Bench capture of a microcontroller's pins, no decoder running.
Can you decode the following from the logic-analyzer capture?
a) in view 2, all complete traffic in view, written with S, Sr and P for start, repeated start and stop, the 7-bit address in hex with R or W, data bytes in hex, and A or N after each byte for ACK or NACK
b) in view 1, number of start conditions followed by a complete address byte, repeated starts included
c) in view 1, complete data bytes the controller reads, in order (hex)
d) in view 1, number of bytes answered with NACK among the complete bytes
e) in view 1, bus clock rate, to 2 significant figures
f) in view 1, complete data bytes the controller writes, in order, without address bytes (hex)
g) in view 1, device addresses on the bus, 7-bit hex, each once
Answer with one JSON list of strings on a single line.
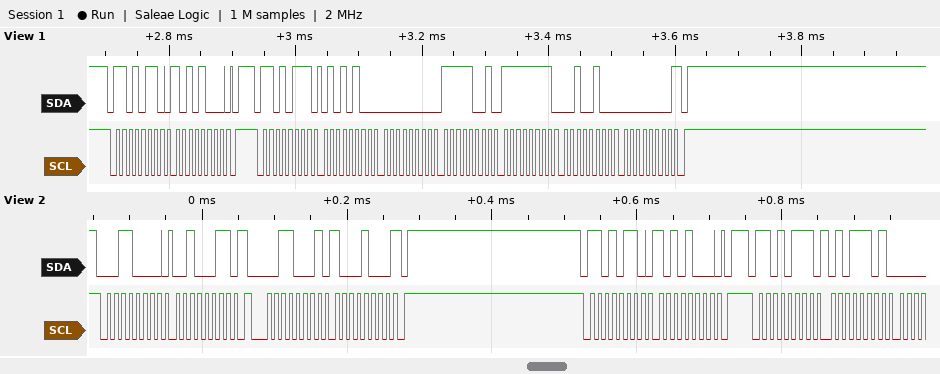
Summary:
["S 18W A 23 A Sr 18R A 88 N P S 6BW A A8 A P S 6BR A 5D A", "2", "54 00 F9 FF 24 00", "1", "100 kHz", "A8", "0x6B"]
